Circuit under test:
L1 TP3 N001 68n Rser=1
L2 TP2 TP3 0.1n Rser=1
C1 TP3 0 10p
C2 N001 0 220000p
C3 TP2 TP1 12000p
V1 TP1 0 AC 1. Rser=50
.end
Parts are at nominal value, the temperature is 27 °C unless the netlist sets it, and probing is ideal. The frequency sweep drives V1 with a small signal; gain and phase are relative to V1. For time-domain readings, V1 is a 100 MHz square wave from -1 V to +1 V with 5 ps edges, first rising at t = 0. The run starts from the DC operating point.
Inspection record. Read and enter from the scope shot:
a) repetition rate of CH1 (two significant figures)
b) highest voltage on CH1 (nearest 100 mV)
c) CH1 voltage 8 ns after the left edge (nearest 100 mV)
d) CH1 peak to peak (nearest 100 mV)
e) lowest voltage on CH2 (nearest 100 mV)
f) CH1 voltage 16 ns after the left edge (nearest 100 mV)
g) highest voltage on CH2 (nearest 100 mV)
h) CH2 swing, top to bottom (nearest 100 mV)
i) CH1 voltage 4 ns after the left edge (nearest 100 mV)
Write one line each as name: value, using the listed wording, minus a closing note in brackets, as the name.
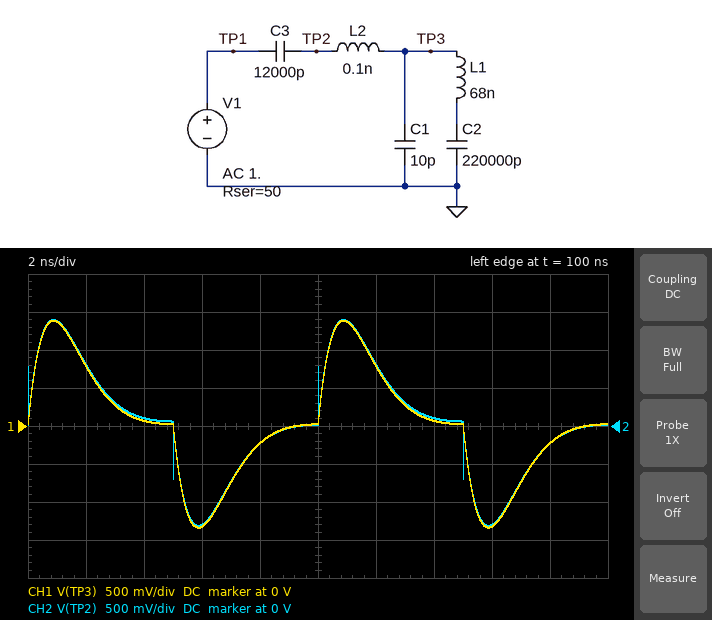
repetition rate of CH1: 100 MHz
highest voltage on CH1: 1.4 V
CH1 voltage 8 ns after the left edge: -200 mV
CH1 peak to peak: 2.7 V
lowest voltage on CH2: -1.3 V
CH1 voltage 16 ns after the left edge: -1.3 V
highest voltage on CH2: 1.4 V
CH2 swing, top to bottom: 2.7 V
CH1 voltage 4 ns after the left edge: 100 mV
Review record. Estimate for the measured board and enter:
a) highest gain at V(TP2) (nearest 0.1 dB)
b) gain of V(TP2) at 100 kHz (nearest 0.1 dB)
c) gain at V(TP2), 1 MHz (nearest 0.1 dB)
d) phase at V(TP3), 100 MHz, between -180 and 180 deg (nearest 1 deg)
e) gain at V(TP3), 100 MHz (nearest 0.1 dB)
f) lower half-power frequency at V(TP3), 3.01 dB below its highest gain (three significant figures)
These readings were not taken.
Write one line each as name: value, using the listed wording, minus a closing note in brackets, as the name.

highest gain at V(TP2): -0.1 dB
gain of V(TP2) at 100 kHz: -26.0 dB
gain at V(TP2), 1 MHz: -28.5 dB
phase at V(TP3), 100 MHz, between -180 and 180 deg: 40 deg
gain at V(TP3), 100 MHz: -2.6 dB
lower half-power frequency at V(TP3), 3.01 dB below its highest gain: 93.1 MHz
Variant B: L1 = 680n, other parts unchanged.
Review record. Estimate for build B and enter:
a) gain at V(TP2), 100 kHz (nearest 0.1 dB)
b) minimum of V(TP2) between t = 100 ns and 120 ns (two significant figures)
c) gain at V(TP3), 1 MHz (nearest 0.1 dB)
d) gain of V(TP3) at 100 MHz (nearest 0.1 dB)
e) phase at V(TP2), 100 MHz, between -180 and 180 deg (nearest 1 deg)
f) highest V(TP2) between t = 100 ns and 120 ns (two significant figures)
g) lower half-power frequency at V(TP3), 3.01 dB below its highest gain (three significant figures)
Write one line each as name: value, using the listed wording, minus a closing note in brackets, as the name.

gain at V(TP2), 100 kHz: -26.4 dB
minimum of V(TP2) between t = 100 ns and 120 ns: -1.0 V
gain at V(TP3), 1 MHz: -23.1 dB
gain of V(TP3) at 100 MHz: -0.2 dB
phase at V(TP2), 100 MHz, between -180 and 180 deg: -11 deg
highest V(TP2) between t = 100 ns and 120 ns: 1.1 V
lower half-power frequency at V(TP3), 3.01 dB below its highest gain: 11.5 MHz
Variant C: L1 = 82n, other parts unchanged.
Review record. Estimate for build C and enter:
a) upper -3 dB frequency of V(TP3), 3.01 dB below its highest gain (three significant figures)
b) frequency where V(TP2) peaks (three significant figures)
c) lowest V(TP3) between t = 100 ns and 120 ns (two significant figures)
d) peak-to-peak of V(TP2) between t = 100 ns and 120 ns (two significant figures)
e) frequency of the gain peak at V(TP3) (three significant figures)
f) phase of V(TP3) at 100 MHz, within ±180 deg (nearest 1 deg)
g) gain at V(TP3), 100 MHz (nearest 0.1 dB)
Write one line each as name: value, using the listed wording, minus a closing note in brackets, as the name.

upper -3 dB frequency of V(TP3), 3.01 dB below its highest gain: 395 MHz
frequency where V(TP2) peaks: 177 MHz
lowest V(TP3) between t = 100 ns and 120 ns: -1.4 V
peak-to-peak of V(TP2) between t = 100 ns and 120 ns: 2.8 V
frequency of the gain peak at V(TP3): 178 MHz
phase of V(TP3) at 100 MHz, within ±180 deg: 33 deg
gain at V(TP3), 100 MHz: -1.7 dB
